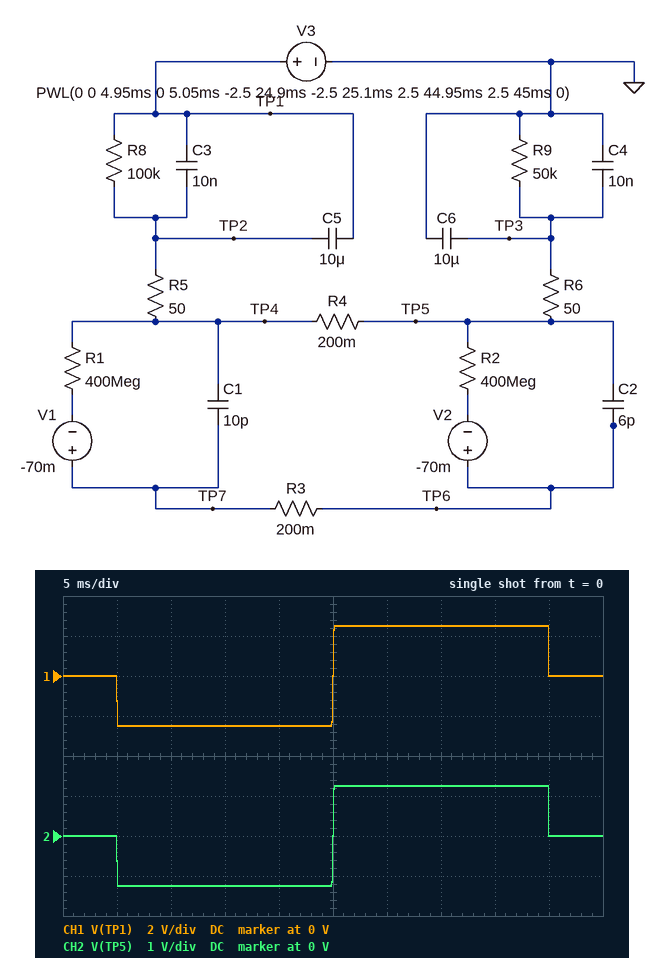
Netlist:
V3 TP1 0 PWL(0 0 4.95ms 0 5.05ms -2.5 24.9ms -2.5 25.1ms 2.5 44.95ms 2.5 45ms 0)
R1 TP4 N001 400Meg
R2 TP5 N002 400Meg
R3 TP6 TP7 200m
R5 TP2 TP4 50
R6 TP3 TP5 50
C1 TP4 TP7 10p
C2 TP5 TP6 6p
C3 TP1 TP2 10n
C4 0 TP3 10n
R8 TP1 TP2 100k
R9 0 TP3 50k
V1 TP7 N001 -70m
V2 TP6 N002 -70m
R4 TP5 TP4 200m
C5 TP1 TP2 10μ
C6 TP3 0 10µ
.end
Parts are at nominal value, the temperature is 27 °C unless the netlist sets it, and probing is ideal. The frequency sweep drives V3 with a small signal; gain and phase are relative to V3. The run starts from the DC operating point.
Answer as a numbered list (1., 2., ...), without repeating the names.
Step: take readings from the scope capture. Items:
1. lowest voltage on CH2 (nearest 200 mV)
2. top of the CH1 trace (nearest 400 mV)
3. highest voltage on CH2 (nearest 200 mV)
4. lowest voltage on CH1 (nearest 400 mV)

1. -1.2 V
2. 2.4 V
3. 1.2 V
4. -2.4 V
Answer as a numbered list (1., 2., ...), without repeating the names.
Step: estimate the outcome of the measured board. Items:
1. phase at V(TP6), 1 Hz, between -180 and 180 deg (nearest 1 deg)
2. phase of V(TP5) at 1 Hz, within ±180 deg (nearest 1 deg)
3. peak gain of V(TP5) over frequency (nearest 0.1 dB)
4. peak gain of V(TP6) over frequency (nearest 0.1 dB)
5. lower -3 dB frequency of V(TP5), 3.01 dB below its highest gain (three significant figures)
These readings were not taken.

1. 4 deg
2. 4 deg
3. -6.0 dB
4. -6.0 dB
5. 79.4 mHz
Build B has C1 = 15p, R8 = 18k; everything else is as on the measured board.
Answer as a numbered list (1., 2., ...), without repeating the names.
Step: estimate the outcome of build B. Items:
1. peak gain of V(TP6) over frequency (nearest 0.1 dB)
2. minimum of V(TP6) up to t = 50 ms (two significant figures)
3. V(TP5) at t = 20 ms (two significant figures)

1. -2.7 dB
2. -1.4 V
3. -1.3 V
